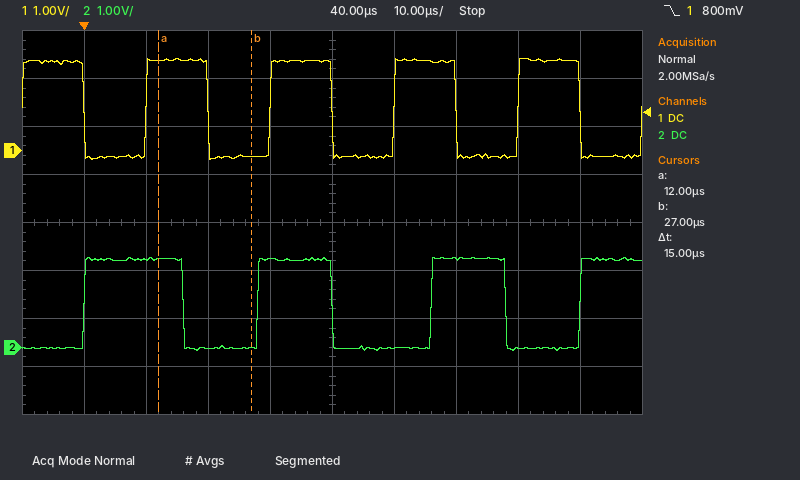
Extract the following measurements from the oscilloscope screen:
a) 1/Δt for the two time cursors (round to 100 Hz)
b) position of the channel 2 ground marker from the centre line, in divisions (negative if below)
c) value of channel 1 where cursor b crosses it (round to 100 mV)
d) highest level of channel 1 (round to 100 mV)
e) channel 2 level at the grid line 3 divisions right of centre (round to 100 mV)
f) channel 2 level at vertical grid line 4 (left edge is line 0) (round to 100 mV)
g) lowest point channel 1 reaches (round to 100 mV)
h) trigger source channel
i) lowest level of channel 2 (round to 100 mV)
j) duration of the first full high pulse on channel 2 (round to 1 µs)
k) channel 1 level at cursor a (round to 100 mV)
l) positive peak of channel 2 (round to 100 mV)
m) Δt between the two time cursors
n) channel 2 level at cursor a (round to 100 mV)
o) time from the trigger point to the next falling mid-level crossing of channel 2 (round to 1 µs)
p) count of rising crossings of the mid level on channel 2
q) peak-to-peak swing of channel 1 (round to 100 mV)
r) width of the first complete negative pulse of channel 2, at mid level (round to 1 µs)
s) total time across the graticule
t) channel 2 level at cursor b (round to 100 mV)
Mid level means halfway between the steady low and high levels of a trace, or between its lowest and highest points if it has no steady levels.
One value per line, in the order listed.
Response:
66.7 kHz
-2.6 div
-100 mV
1.9 V
0.0 V
1.8 V
-200 mV
channel 1
-100 mV
16 µs
1.9 V
1.9 V
15 µs
1.8 V
16 µs
4
2.1 V
12 µs
100 µs
0.0 V
